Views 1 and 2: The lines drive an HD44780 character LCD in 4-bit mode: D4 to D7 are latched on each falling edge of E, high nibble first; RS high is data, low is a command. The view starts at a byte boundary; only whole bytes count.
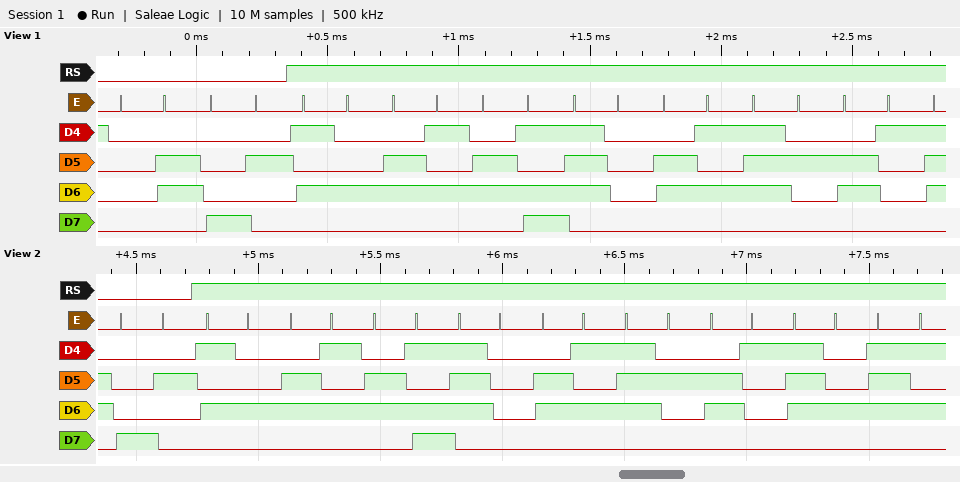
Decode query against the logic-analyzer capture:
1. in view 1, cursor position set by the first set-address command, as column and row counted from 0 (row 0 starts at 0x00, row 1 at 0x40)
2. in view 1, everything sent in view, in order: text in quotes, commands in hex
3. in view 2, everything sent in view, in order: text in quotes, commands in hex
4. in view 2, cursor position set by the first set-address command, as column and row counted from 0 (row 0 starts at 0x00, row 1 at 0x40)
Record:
column 2, row 0
0x06 0x82 "Tempera"
0x82 "Temperatu"
column 2, row 0
